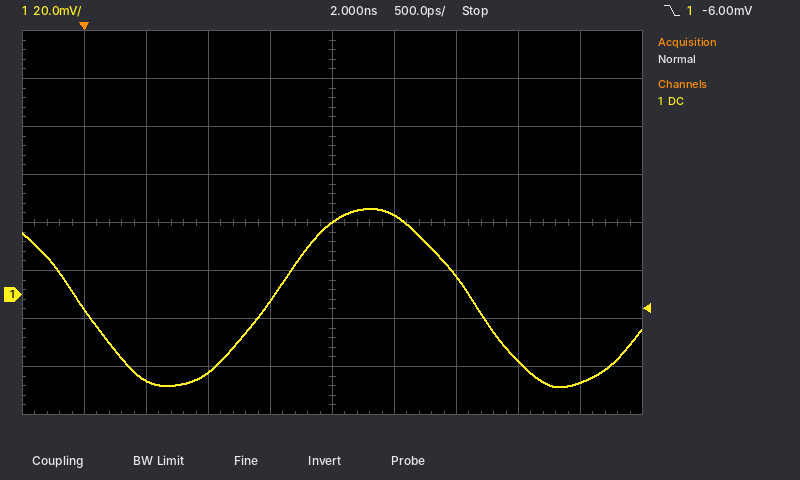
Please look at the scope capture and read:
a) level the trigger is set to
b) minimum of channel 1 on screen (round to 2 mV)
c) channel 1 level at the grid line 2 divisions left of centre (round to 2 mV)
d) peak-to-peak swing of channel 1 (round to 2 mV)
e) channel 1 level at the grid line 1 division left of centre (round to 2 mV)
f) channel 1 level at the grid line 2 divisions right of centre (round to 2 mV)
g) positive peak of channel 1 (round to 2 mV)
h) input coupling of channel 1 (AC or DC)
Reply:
-6.00 mV
-38 mV
-32 mV
74 mV
-2 mV
8 mV
36 mV
DC
